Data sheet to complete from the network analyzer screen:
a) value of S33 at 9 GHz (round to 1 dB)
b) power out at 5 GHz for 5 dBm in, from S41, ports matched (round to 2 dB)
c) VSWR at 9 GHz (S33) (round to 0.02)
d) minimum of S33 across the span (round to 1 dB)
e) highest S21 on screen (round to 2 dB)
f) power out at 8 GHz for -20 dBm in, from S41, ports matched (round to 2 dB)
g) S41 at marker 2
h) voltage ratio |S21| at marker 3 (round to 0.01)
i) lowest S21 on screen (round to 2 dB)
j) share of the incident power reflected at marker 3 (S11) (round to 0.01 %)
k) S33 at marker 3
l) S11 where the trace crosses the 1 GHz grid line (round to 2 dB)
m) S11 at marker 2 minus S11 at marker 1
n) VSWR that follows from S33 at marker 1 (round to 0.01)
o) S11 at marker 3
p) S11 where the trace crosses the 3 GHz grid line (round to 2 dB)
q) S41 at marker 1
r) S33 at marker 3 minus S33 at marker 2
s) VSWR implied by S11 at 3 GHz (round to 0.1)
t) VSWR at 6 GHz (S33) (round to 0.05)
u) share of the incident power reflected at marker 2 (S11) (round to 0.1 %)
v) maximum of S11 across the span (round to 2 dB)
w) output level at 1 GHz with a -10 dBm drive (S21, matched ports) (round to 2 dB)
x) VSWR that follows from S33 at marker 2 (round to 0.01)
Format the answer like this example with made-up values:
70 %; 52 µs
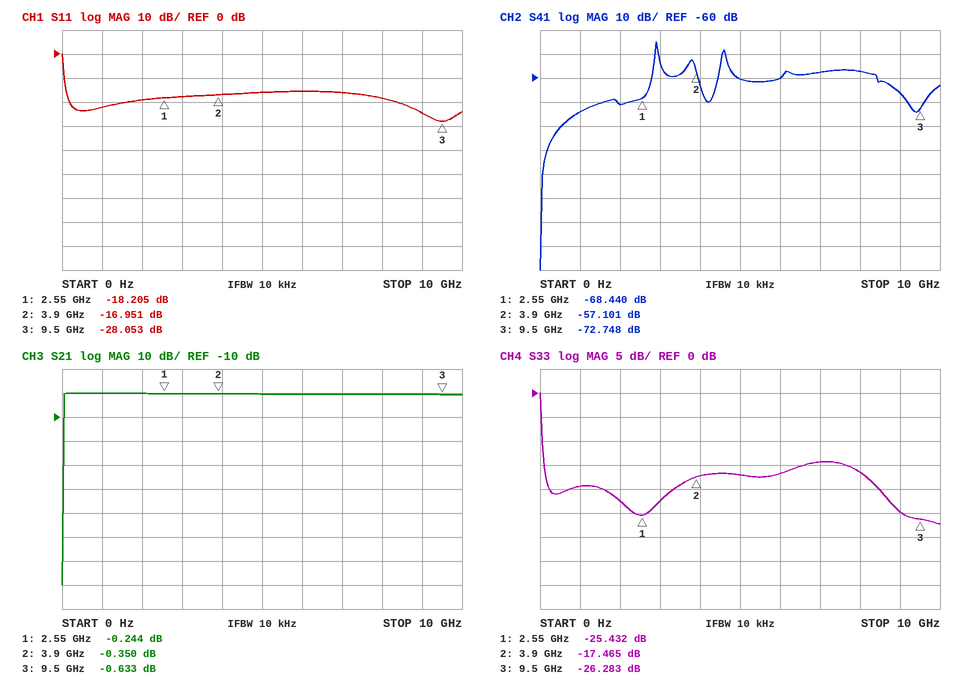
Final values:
-25 dB; -56 dBm; 1.12; -27 dB; 0 dB; -78 dBm; -57.101 dB; 0.93; -80 dB; 0.16 %; -26.283 dB; -22 dB; 1.254 dB; 1.11; -28.053 dB; -18 dB; -68.440 dB; -8.818 dB; 1.3; 1.35; 2.0 %; 0 dB; -10 dBm; 1.31
